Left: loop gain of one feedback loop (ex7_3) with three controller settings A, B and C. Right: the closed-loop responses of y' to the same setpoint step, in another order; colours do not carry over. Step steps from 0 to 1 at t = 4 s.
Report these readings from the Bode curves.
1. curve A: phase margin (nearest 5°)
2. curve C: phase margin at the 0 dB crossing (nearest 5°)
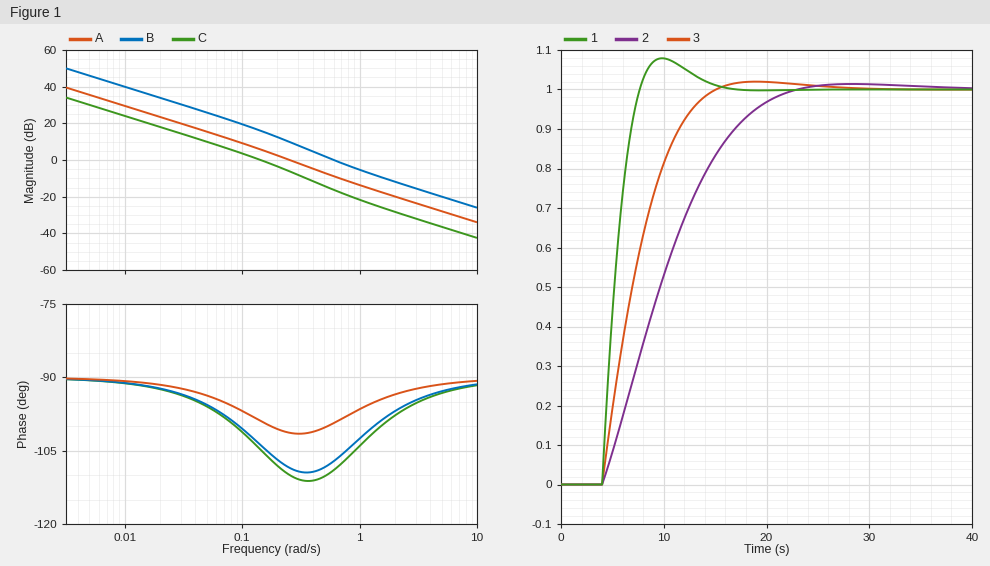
80°
75°
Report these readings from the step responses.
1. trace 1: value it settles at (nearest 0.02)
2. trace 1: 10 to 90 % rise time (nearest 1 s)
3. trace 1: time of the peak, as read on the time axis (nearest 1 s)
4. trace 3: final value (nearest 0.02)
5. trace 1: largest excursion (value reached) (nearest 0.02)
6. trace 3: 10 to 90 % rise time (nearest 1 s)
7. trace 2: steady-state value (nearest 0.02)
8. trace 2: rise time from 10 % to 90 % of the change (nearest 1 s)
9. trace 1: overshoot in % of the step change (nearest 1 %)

1.00
3 s
10 s
1.00
1.08
7 s
1.00
12 s
8 %
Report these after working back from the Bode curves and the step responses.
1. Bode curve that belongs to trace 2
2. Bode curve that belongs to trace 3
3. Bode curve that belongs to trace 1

C
A
B
